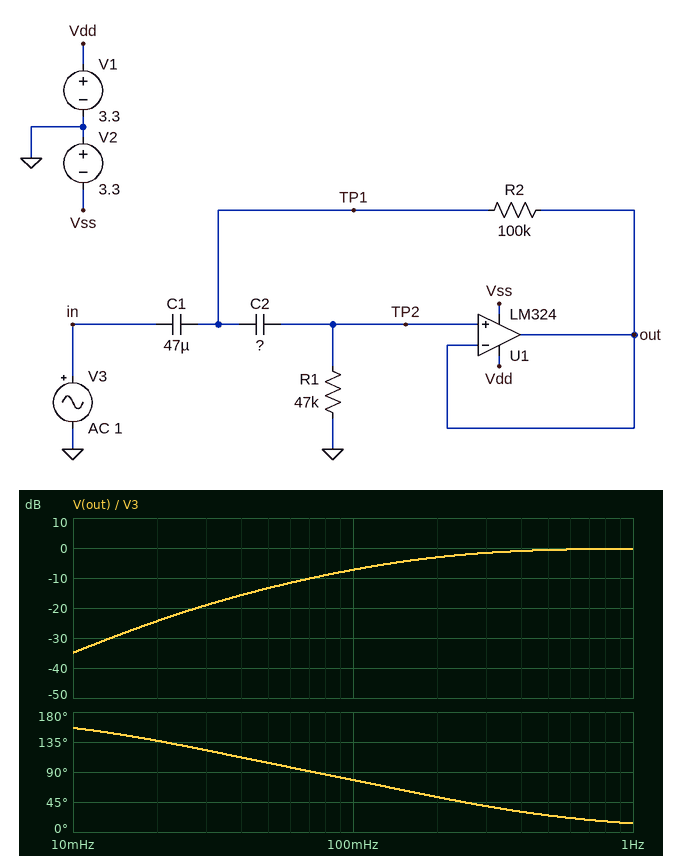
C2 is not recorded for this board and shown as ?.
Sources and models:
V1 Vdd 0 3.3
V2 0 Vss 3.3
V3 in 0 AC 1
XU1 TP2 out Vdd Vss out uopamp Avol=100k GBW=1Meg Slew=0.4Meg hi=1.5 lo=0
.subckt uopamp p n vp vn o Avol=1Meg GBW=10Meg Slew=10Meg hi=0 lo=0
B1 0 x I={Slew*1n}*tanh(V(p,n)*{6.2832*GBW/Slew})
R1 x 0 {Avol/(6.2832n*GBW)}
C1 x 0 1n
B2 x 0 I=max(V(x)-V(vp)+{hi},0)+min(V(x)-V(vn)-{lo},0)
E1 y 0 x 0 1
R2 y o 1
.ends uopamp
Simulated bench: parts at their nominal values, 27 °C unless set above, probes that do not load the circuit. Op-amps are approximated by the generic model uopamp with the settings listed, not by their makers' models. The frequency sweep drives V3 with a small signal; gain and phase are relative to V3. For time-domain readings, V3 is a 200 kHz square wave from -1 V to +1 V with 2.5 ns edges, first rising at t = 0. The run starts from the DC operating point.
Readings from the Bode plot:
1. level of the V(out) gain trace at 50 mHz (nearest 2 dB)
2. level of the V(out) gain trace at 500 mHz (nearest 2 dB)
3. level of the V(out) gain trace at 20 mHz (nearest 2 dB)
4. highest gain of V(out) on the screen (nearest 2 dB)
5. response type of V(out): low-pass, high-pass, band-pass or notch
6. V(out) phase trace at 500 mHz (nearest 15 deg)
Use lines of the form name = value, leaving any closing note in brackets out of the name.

level of the V(out) gain trace at 50 mHz = -14 dB
level of the V(out) gain trace at 500 mHz = 0 dB
level of the V(out) gain trace at 20 mHz = -24 dB
highest gain of V(out) on the screen = 0 dB
response type of V(out): low-pass, high-pass, band-pass or notch = high-pass
V(out) phase trace at 500 mHz = 30 deg
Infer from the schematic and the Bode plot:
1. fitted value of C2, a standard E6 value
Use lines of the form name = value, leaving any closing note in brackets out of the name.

fitted value of C2, a standard E6 value = 22 µF
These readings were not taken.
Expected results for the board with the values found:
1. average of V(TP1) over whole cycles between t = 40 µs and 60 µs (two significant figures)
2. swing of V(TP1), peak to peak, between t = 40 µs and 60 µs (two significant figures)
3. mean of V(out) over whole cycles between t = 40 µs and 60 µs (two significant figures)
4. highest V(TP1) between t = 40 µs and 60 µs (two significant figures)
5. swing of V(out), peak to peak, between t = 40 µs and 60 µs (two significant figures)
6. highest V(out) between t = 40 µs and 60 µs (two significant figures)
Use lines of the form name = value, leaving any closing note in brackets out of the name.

average of V(TP1) over whole cycles between t = 40 µs and 60 µs = 1.0 V
swing of V(TP1), peak to peak, between t = 40 µs and 60 µs = 2.0 V
mean of V(out) over whole cycles between t = 40 µs and 60 µs = 600 mV
highest V(TP1) between t = 40 µs and 60 µs = 2.0 V
swing of V(out), peak to peak, between t = 40 µs and 60 µs = 1.0 V
highest V(out) between t = 40 µs and 60 µs = 1.1 V
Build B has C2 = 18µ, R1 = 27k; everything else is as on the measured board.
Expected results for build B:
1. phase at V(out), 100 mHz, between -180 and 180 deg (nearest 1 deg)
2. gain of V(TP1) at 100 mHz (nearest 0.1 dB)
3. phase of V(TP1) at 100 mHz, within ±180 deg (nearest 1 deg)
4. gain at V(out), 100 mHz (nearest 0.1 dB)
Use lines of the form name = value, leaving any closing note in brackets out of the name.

phase at V(out), 100 mHz, between -180 and 180 deg = 91 deg
gain of V(TP1) at 100 mHz = -2.4 dB
phase of V(TP1) at 100 mHz, within ±180 deg = 18 deg
gain at V(out), 100 mHz = -13.1 dB
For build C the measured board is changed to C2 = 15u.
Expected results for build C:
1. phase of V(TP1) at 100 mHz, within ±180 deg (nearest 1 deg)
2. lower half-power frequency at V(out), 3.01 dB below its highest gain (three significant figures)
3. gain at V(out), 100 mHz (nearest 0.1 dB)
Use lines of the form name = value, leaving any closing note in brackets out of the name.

phase of V(TP1) at 100 mHz, within ±180 deg = 19 deg
lower half-power frequency at V(out), 3.01 dB below its highest gain = 272 mHz
gain at V(out), 100 mHz = -9.5 dB
